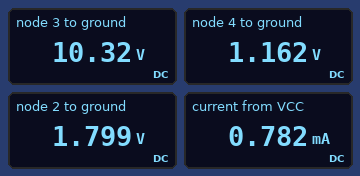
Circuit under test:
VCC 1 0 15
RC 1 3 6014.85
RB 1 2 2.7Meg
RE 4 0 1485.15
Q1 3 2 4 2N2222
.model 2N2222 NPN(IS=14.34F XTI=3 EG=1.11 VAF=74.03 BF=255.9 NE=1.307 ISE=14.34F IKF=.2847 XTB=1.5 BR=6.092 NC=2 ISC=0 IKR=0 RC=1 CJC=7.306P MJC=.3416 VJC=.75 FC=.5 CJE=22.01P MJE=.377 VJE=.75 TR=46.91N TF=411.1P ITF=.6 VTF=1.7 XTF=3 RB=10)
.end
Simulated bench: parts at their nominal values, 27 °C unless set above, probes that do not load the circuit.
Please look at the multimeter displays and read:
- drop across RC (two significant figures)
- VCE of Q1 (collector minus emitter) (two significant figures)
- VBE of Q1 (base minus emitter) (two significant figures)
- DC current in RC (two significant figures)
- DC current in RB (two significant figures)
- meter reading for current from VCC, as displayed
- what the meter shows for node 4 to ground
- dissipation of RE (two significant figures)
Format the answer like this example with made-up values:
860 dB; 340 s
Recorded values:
4.7 V; 9.2 V; 640 mV; 780 µA; 4.9 µA; 0.782 mA; 1.162 V; 910 µW
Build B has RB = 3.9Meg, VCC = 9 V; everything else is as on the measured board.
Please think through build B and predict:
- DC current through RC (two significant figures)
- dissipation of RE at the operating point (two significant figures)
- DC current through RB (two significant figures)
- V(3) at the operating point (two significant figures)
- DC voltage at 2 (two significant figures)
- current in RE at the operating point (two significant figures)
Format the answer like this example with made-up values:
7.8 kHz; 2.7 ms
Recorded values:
280 µA; 120 µW; 2.0 µA; 7.3 V; 1.0 V; 290 µA
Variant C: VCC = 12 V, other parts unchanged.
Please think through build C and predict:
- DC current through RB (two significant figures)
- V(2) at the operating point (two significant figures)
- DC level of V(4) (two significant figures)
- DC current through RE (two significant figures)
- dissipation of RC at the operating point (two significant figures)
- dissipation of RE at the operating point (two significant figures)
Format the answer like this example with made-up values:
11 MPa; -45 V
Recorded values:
3.9 µA; 1.5 V; 880 mV; 590 µA; 2.1 mW; 520 µW
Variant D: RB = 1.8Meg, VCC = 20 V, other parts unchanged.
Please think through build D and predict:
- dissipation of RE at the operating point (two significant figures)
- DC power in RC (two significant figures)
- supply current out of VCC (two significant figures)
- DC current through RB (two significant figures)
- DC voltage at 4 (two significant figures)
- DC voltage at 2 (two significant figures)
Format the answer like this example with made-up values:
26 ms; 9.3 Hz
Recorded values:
3.8 mW; 15 mW; 1.6 mA; 9.4 µA; 2.4 V; 3.0 V
